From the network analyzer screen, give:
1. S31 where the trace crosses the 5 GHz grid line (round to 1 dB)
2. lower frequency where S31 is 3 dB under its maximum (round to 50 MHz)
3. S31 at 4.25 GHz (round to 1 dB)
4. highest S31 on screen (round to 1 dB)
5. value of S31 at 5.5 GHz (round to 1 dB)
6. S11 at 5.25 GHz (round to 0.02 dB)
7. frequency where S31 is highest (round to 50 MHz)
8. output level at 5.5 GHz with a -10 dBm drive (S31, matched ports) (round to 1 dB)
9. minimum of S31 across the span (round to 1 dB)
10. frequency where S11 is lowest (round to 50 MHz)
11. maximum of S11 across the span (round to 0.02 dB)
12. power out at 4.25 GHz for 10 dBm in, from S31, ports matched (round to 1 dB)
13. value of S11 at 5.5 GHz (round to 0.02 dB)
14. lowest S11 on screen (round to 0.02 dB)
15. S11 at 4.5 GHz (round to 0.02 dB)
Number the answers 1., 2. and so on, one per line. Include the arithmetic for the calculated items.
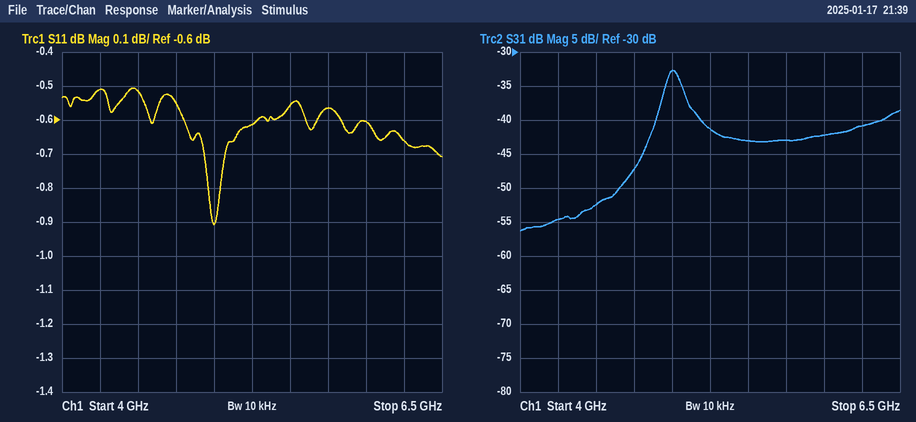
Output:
1. -33 dB
2. 4.95 GHz
3. -55 dB
4. -33 dB
5. -43 dB
6. -0.62 dB
7. 5.00 GHz
8. -10 dBm + (-43 dB) = -53 dBm
9. -56 dB
10. 5.00 GHz
11. -0.50 dB
12. 10 dBm + (-55 dB) = -45 dBm
13. -0.56 dB
14. -0.90 dB
15. -0.52 dB
